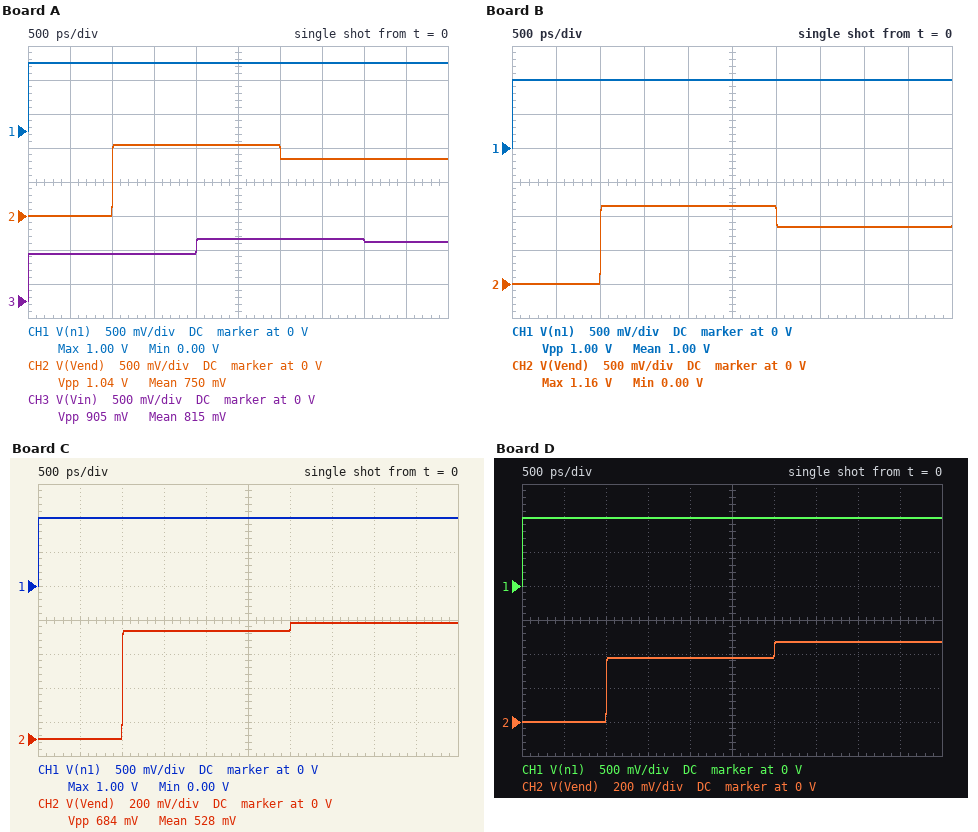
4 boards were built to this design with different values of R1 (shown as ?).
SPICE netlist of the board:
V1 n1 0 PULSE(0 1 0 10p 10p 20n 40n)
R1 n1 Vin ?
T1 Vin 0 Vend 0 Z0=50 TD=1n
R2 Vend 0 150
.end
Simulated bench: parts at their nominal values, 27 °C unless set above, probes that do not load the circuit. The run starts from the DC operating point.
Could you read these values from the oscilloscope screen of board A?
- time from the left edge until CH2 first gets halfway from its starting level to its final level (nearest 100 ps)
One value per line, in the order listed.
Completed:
1.0 ns
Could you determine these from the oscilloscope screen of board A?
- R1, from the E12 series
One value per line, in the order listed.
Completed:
22 Ω
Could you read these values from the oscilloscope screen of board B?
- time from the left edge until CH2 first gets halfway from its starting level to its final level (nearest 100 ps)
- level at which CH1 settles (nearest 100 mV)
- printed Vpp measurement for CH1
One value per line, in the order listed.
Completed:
1.0 ns
1.0 V
1.00 V
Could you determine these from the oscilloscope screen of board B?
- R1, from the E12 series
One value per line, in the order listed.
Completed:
15 Ω
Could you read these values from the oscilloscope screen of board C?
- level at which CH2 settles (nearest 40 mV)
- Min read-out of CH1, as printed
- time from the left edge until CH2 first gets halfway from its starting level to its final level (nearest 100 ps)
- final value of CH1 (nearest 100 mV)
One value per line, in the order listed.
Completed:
680 mV
0.00 V
1.0 ns
1.0 V
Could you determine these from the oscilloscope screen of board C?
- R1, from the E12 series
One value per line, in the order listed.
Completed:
68 Ω
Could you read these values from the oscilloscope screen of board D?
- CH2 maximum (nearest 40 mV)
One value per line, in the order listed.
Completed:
480 mV
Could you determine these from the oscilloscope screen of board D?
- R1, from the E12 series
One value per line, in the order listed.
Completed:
150 Ω
